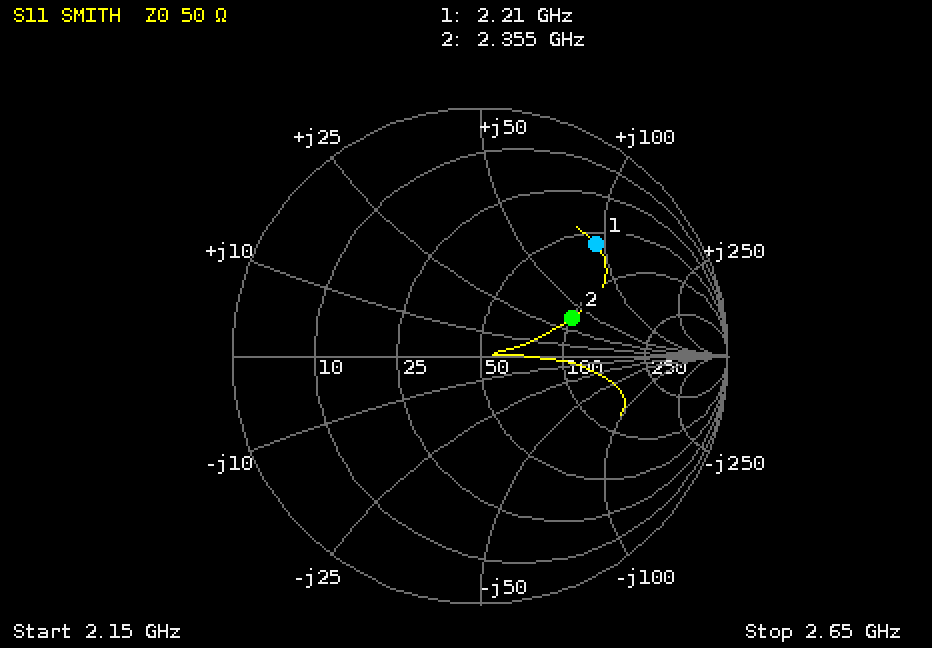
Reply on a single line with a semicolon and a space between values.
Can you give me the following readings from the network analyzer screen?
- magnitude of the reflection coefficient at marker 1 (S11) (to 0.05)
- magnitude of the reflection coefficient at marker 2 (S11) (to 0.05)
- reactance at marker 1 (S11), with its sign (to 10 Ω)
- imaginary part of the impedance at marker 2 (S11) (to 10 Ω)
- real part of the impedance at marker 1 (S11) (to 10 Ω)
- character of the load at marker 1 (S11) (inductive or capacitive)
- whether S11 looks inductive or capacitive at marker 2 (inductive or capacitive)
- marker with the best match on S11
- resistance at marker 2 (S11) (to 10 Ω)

0.65; 0.40; +90 Ω; +40 Ω; 60 Ω; inductive; inductive; marker 2; 100 Ω
